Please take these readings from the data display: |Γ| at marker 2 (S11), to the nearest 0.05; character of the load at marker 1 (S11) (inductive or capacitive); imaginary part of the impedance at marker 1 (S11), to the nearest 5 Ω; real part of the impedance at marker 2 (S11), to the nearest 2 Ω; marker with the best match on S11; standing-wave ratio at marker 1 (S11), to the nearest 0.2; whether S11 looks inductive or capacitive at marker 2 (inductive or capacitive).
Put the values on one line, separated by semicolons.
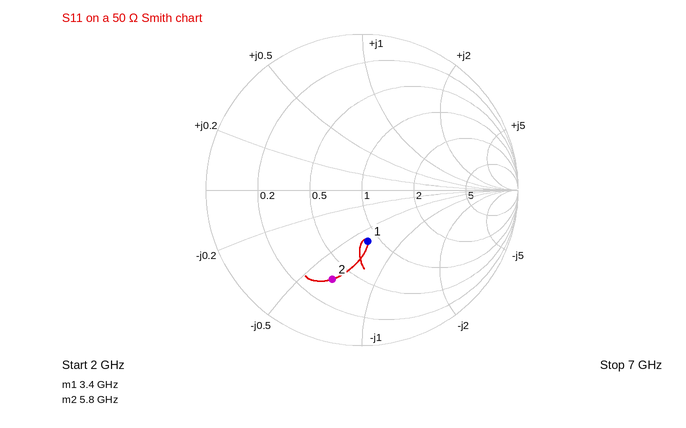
0.60; capacitive; -30 Ω; 18 Ω; marker 1; 2.0; capacitive
